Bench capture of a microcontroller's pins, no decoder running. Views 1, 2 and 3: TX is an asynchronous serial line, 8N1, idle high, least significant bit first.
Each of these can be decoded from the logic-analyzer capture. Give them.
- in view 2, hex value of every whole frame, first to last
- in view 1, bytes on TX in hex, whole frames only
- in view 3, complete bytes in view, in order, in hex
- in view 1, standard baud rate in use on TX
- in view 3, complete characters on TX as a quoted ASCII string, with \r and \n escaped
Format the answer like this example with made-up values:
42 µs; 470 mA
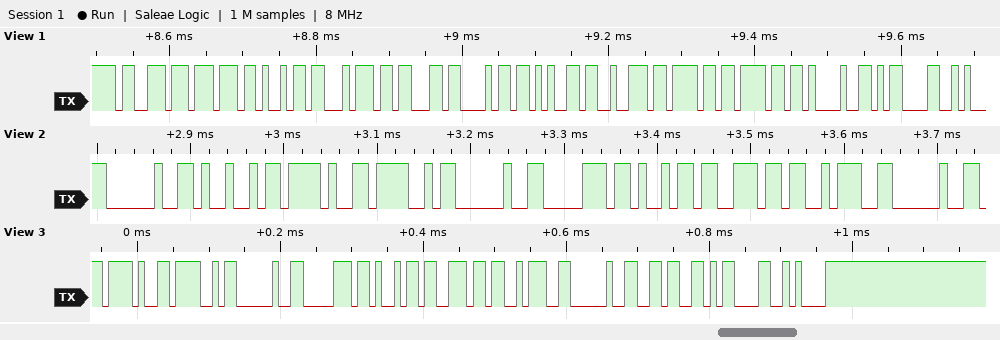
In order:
0x20 0x49 0x2F 0x4F 0x20 0x70 0x69 0x6E 0x3A 0x20; 0x73 0x77 0x69 0x74 0x63 0x68 0x65 0x72 0x6F 0x6F 0x21 0x0D; 0x2F 0x4F 0x20 0x70 0x69 0x6E 0x3A 0x20 0x36 0x0D 0x0A; 115200 baud; "/O pin: 6\r\n"
